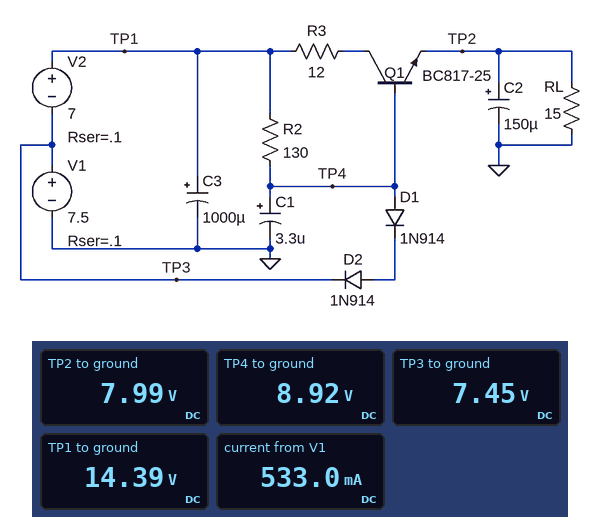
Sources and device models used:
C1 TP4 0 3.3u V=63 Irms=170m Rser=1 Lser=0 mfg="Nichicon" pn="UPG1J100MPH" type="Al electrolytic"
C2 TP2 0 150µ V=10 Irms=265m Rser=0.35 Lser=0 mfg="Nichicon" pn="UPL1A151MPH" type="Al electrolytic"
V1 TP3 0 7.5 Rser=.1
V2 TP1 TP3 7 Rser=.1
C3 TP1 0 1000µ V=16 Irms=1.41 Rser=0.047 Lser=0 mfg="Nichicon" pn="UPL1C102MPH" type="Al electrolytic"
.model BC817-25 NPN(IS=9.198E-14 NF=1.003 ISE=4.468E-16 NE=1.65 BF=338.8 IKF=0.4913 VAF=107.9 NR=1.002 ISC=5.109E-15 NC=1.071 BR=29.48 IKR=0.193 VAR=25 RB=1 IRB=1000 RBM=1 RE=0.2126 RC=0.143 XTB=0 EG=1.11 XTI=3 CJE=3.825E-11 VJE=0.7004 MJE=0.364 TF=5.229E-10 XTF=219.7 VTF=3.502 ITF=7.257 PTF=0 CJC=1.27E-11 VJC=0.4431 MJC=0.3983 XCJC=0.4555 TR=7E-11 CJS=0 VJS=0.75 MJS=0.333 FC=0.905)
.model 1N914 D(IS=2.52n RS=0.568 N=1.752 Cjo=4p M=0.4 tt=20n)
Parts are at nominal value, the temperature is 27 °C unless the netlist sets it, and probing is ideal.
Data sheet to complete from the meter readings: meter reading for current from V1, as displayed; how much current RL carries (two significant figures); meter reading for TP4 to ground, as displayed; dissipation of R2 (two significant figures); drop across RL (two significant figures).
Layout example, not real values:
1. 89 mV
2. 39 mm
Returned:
1. 533.0 mA
2. 530 mA
3. 8.92 V
4. 230 mW
5. 8.0 V
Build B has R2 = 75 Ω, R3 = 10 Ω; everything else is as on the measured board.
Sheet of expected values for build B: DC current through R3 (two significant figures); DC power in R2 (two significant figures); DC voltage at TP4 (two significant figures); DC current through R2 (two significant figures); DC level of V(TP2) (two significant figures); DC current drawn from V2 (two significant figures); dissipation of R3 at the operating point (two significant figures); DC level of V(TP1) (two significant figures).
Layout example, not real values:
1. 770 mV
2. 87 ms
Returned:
1. 540 mA
2. 380 mW
3. 9.1 V
4. 71 mA
5. 8.2 V
6. 610 mA
7. 2.9 W
8. 14 V
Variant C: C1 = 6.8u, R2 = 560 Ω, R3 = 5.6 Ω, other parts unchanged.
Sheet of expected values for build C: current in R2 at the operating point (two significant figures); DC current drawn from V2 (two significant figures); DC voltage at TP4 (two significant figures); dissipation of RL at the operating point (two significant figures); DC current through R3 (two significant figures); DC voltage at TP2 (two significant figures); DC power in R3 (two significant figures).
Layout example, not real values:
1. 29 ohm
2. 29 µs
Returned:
1. 10 mA
2. 530 mA
3. 8.8 V
4. 4.2 W
5. 520 mA
6. 7.9 V
7. 1.5 W
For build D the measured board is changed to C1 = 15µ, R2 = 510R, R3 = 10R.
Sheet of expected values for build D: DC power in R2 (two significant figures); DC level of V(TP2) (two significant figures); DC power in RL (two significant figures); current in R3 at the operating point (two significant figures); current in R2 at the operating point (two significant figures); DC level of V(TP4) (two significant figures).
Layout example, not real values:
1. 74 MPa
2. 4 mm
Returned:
1. 61 mW
2. 7.9 V
3. 4.2 W
4. 520 mA
5. 11 mA
6. 8.8 V
